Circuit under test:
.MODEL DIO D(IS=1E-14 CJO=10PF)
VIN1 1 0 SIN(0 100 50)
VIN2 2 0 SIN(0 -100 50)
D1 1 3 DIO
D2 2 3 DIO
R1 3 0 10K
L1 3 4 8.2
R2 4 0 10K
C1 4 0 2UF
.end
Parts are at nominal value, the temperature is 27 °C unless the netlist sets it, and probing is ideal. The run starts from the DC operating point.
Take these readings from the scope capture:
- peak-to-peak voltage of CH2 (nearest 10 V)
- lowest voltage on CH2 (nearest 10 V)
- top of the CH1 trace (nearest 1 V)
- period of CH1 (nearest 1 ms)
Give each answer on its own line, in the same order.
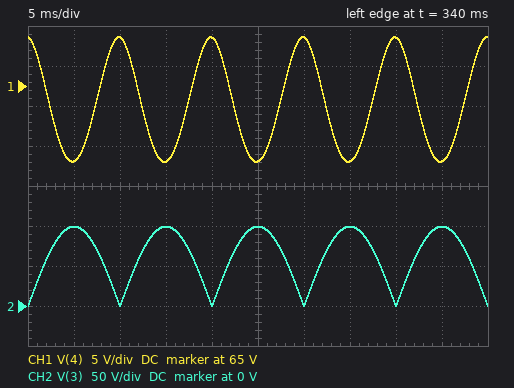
100 V
0 V
71 V
10 ms
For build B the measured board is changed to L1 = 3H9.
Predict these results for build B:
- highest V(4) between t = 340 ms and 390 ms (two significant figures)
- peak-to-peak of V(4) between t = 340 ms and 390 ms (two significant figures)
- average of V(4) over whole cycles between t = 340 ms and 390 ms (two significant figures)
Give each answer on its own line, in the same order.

87 V
29 V
72 V
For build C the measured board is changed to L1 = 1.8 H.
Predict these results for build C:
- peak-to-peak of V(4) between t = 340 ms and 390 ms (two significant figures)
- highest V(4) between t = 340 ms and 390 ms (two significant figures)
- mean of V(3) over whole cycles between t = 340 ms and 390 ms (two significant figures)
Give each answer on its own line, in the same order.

41 V
110 V
84 V
